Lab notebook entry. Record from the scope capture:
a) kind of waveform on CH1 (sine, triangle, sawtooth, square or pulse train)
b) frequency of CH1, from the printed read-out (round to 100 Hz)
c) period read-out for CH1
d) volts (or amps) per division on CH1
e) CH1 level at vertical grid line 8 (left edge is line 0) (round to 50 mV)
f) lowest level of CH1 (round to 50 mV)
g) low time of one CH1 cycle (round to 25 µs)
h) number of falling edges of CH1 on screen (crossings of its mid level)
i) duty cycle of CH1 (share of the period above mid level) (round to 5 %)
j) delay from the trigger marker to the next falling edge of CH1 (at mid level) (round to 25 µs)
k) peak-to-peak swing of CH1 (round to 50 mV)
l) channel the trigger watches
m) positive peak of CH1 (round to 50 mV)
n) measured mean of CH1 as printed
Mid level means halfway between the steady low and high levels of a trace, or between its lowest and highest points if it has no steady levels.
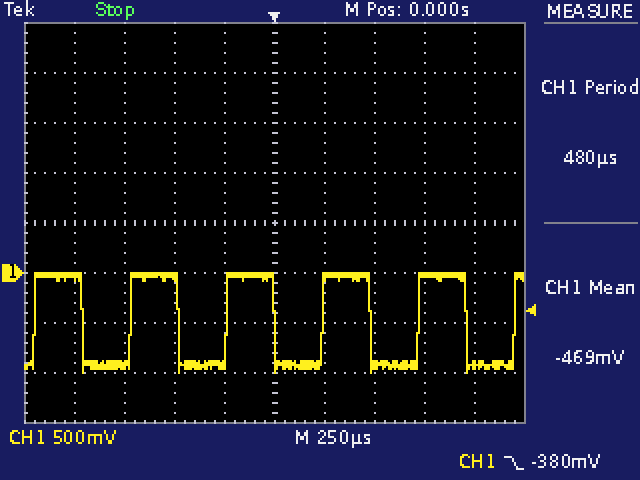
square
2.1 kHz
480 µs
500 mV
0 mV
-1.00 V
250 µs
5
50 %
475 µs
1.00 V
CH1
0 mV
-469 mV
